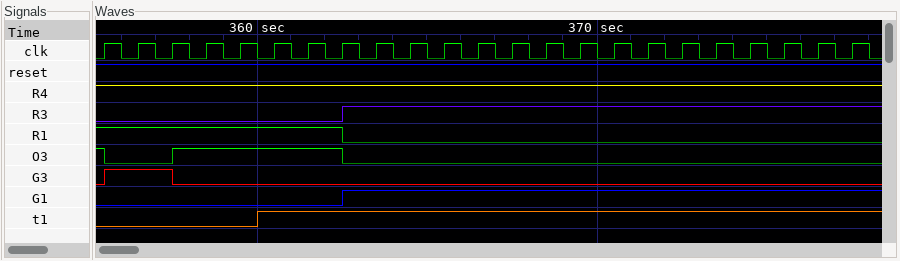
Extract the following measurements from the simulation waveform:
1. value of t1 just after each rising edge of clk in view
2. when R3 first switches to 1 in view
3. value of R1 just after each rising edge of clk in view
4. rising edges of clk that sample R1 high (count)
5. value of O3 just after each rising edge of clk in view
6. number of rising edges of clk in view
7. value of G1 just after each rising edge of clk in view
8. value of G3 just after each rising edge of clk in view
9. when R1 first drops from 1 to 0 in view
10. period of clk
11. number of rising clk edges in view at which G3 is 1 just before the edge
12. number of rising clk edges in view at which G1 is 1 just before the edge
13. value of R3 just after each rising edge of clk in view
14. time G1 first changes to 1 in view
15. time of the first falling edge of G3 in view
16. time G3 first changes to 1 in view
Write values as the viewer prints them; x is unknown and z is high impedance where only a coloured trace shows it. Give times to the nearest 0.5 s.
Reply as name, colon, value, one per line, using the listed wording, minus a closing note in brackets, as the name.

value of t1 just after each rising edge of clk in view: 0 0 0 0 0 1 1 1 1 1 1 1 1 1 1 1 1 1 1 1 1 1 1
when R3 first switches to 1 in view: 362.5 s
value of R1 just after each rising edge of clk in view: 1 1 1 1 1 1 1 0 0 0 0 0 0 0 0 0 0 0 0 0 0 0 0
rising edges of clk that sample R1 high: 8
value of O3 just after each rising edge of clk in view: 0 0 1 1 1 1 1 0 0 0 0 0 0 0 0 0 0 0 0 0 0 0 0
number of rising edges of clk in view: 23
value of G1 just after each rising edge of clk in view: 0 0 0 0 0 0 0 1 1 1 1 1 1 1 1 1 1 1 1 1 1 1 1
value of G3 just after each rising edge of clk in view: 1 1 0 0 0 0 0 0 0 0 0 0 0 0 0 0 0 0 0 0 0 0 0
when R1 first drops from 1 to 0 in view: 362.5 s
period of clk: 1 s
number of rising clk edges in view at which G3 is 1 just before the edge: 2
number of rising clk edges in view at which G1 is 1 just before the edge: 15
value of R3 just after each rising edge of clk in view: 0 0 0 0 0 0 0 1 1 1 1 1 1 1 1 1 1 1 1 1 1 1 1
time G1 first changes to 1 in view: 362.5 s
time of the first falling edge of G3 in view: 357.5 s
time G3 first changes to 1 in view: 355.5 s
